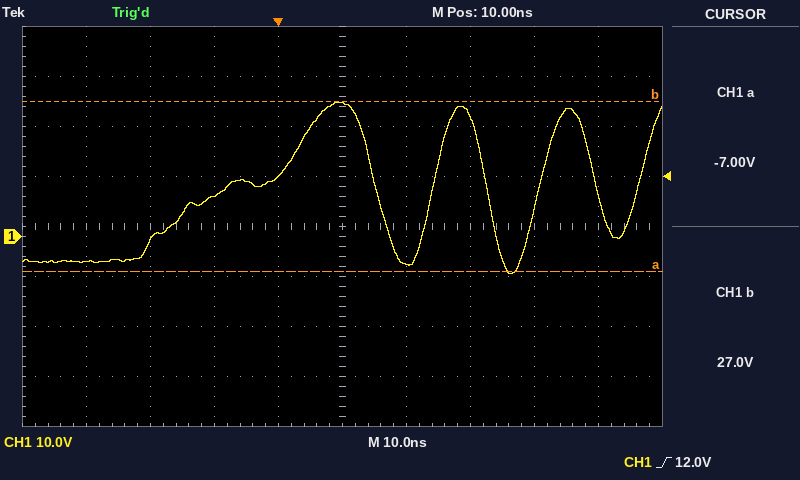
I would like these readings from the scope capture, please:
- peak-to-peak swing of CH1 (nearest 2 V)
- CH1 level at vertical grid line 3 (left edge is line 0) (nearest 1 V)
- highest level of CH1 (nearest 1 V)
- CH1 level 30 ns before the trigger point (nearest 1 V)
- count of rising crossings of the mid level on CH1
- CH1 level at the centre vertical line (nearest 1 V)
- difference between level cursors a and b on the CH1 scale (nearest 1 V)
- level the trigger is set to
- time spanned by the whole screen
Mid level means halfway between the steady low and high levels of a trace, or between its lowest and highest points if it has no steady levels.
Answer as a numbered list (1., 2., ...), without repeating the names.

1. 34 V
2. 8 V
3. 27 V
4. -5 V
5. 4
6. 27 V
7. 34 V
8. 12.0 V
9. 100 ns
